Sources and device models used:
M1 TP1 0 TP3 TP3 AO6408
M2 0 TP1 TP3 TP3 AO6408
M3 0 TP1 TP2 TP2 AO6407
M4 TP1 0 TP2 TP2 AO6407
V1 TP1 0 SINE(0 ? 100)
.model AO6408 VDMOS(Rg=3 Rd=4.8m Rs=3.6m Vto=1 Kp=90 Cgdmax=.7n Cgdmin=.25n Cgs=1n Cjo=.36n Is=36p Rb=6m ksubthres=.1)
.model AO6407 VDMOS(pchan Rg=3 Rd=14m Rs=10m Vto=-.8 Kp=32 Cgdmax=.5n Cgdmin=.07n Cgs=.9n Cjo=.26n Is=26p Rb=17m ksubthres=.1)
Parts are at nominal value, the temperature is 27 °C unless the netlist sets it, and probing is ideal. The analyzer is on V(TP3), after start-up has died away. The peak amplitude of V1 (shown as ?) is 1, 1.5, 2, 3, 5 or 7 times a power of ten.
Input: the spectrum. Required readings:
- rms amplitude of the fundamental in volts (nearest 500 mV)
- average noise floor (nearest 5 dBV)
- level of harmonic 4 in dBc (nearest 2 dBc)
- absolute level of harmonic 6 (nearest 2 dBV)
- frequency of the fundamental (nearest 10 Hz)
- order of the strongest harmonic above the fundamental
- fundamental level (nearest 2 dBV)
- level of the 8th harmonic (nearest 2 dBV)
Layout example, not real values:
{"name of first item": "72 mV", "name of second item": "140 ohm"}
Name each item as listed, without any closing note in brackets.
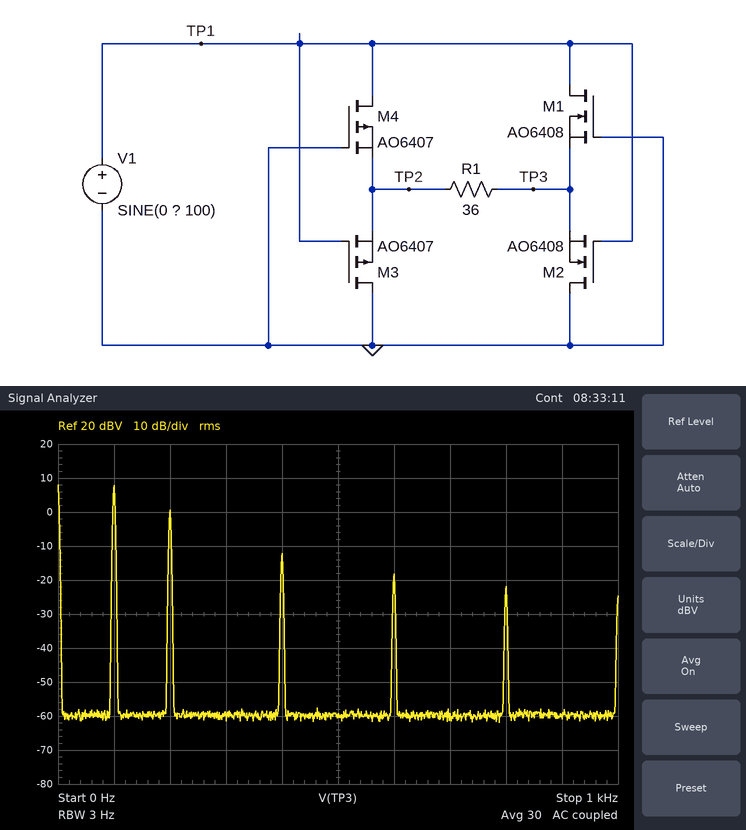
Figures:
{"rms amplitude of the fundamental in volts": "2.5 V", "average noise floor": "-60 dBV", "level of harmonic 4 in dBc": "-20 dBc", "absolute level of harmonic 6": "-18 dBV", "frequency of the fundamental": "100 Hz", "order of the strongest harmonic above the fundamental": "2", "fundamental level": "8 dBV", "level of the 8th harmonic": "-22 dBV"}
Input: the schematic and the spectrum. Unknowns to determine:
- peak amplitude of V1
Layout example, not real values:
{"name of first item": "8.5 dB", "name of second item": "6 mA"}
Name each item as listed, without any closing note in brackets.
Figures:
{"peak amplitude of V1": "7 V"}
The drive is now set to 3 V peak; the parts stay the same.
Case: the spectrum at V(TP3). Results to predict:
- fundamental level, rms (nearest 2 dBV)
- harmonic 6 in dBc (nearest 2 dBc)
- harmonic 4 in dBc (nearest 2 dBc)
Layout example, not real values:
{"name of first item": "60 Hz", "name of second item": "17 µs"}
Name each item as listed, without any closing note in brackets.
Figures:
{"fundamental level, rms": "0 dBV", "harmonic 6 in dBc": "-22 dBc", "harmonic 4 in dBc": "-16 dBc"}
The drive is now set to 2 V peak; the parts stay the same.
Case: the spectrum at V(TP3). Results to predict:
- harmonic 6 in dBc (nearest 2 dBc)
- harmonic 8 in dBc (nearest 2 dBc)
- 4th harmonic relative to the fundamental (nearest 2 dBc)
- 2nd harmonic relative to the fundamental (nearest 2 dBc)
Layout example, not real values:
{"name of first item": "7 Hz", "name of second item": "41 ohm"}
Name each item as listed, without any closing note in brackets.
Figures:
{"harmonic 6 in dBc": "-30 dBc", "harmonic 8 in dBc": "-26 dBc", "4th harmonic relative to the fundamental": "-16 dBc", "2nd harmonic relative to the fundamental": "-4 dBc"}
